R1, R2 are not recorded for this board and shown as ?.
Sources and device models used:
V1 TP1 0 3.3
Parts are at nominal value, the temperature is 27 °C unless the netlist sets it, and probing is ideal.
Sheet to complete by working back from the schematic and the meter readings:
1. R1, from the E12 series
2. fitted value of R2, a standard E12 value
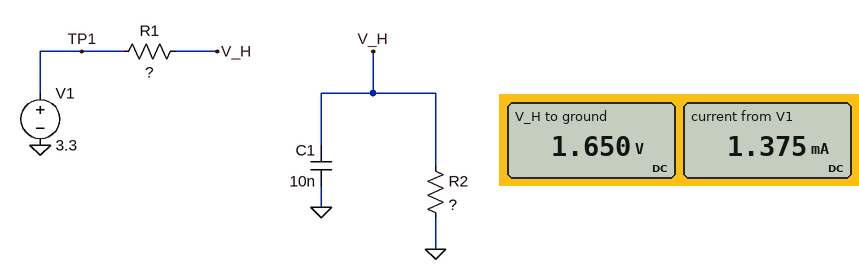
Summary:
1.2 kΩ
1.2 kΩ
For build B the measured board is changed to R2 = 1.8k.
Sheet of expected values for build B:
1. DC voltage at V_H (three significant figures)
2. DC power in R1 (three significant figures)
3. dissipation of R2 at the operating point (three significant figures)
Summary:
1.98 V
1.45 mW
2.18 mW
